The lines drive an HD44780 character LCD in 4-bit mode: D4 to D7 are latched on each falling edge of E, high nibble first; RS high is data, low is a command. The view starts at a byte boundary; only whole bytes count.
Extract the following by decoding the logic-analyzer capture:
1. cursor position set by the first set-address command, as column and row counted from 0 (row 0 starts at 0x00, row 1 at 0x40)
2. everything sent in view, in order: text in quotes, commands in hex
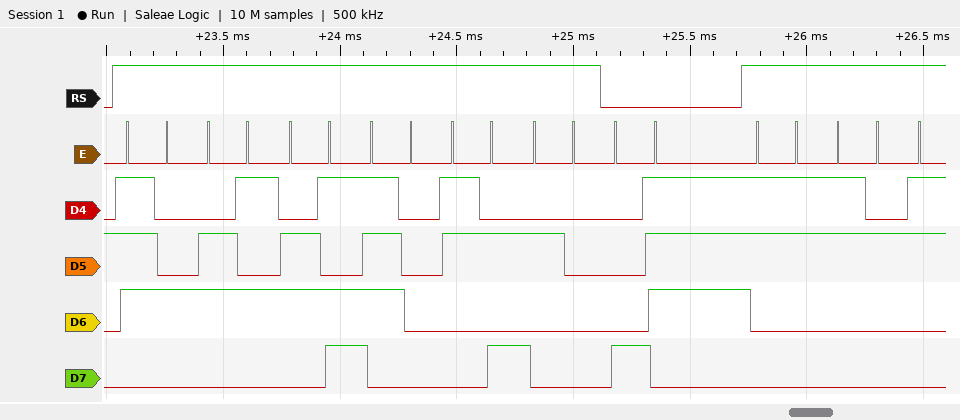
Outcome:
column 7, row 0
"temp: " 0x87 "32"
